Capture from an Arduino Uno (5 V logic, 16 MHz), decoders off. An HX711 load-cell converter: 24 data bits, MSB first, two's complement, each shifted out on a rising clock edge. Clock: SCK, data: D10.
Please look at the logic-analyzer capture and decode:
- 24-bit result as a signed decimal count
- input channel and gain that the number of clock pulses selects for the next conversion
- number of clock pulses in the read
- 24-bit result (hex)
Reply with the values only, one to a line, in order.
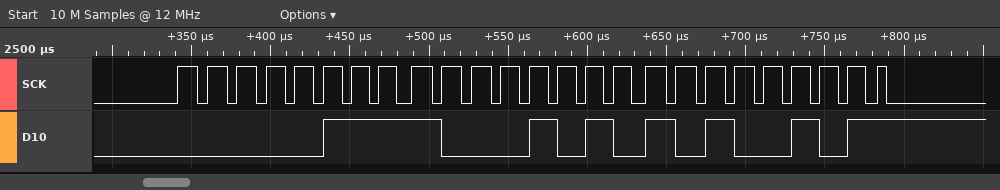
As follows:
494245
channel A, gain 128
25
0x078AA5
